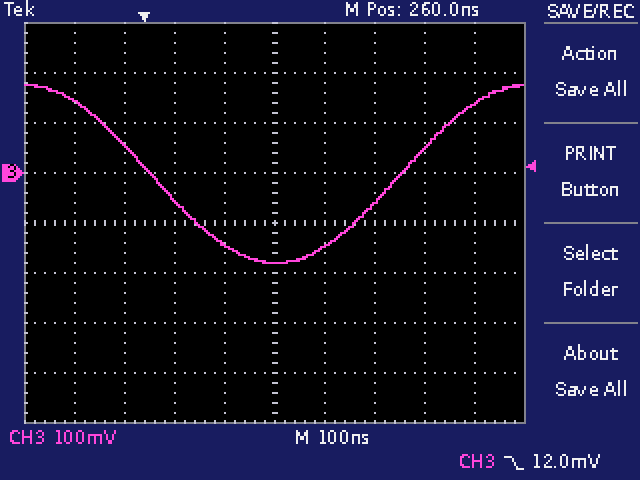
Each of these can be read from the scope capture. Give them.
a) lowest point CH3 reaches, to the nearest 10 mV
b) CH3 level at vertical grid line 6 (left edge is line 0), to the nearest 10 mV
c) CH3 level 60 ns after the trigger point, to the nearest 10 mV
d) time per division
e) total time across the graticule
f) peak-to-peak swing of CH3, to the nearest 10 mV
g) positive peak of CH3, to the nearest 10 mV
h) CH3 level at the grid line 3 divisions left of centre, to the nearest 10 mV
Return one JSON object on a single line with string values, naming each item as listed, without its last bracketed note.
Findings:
{"lowest point CH3 reaches, to the nearest 10 mV": "-180 mV", "CH3 level at vertical grid line 6 (left edge is line 0), to the nearest 10 mV": "-150 mV", "CH3 level 60 ns after the trigger point, to the nearest 10 mV": "-50 mV", "time per division": "100 ns", "total time across the graticule": "1 µs", "peak-to-peak swing of CH3, to the nearest 10 mV": "360 mV", "positive peak of CH3, to the nearest 10 mV": "180 mV", "CH3 level at the grid line 3 divisions left of centre, to the nearest 10 mV": "60 mV"}
